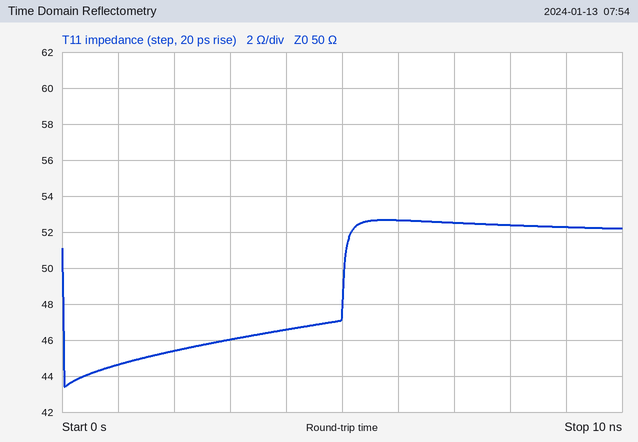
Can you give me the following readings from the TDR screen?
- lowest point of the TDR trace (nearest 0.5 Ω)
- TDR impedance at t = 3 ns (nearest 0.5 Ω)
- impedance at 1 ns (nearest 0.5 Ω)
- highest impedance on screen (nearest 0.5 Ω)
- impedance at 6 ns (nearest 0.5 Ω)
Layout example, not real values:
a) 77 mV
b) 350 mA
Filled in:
a) 43.5 Ω
b) 46.0 Ω
c) 44.5 Ω
d) 52.5 Ω
e) 52.5 Ω
